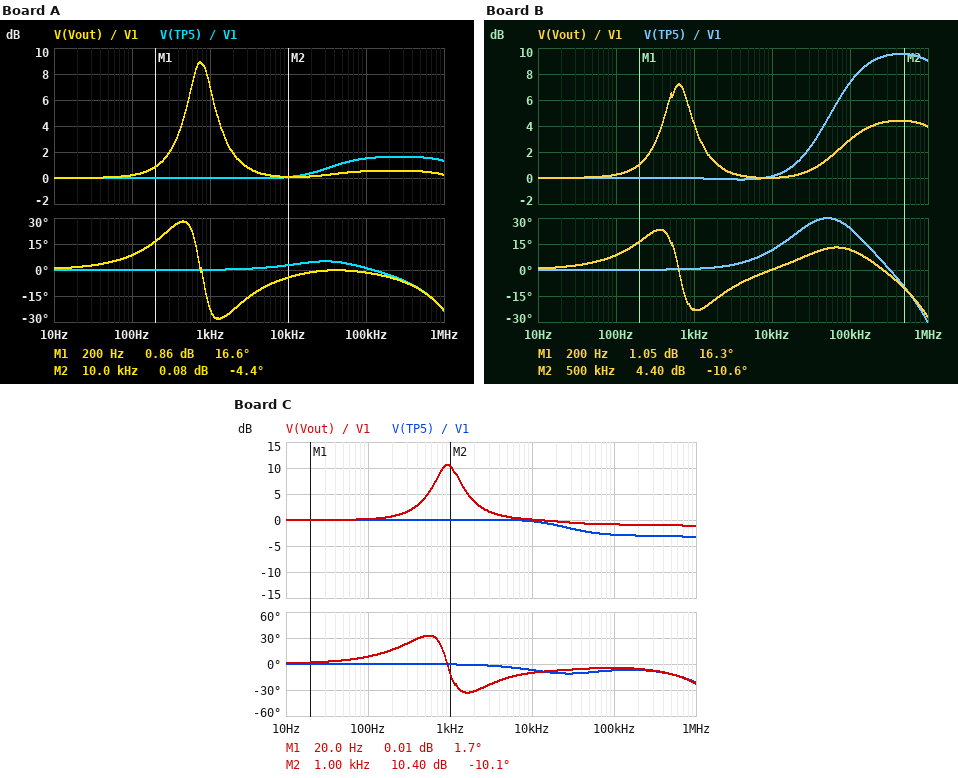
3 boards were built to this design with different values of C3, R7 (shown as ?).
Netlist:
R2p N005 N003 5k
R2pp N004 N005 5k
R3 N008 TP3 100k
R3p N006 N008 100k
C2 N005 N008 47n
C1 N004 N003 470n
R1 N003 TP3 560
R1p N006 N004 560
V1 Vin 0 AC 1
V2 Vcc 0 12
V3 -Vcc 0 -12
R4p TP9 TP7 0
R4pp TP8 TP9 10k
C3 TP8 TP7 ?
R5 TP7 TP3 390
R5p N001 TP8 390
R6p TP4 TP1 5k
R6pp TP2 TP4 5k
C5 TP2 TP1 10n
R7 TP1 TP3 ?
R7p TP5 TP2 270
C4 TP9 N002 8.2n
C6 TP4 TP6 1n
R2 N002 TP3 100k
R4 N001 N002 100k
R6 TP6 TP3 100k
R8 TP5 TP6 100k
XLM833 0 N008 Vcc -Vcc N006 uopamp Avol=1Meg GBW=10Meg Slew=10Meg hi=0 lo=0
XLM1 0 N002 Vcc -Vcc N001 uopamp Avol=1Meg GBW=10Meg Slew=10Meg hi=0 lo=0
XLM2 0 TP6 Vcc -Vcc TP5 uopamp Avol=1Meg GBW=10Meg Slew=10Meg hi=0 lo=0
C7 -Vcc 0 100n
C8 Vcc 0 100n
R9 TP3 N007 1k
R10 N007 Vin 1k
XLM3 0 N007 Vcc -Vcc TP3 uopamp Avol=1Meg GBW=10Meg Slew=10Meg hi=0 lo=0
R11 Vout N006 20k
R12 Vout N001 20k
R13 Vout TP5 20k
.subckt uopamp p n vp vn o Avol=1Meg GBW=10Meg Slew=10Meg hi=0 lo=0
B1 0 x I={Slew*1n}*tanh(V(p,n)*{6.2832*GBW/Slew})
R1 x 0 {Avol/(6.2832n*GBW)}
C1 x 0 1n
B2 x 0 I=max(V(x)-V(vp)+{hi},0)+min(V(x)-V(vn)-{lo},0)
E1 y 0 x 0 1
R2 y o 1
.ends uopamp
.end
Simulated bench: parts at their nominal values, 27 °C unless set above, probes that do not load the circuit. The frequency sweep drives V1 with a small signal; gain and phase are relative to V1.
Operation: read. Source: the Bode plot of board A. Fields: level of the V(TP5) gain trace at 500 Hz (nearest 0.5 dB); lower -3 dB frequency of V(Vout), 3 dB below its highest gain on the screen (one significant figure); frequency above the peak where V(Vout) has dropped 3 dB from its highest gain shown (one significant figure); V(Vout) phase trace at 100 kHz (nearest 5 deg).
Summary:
0 dB
500 Hz
1 kHz
0 deg
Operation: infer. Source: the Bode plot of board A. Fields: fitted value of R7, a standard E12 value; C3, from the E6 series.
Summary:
220 Ω
150 nF
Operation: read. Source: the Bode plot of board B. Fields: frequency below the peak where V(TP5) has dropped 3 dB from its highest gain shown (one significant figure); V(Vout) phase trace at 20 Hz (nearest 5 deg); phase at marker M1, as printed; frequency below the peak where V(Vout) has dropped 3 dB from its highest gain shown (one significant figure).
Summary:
80 kHz
0 deg
16.3 deg
400 Hz
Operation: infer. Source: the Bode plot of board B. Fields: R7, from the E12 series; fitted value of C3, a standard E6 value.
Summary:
82 Ω
220 nF
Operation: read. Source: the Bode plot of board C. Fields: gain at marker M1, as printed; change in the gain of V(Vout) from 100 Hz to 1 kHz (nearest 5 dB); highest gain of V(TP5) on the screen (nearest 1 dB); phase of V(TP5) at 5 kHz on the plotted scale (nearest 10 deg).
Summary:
0.01 dB
10 dB
0 dB
0 deg
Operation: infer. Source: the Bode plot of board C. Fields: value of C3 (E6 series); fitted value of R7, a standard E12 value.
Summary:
100 nF
390 Ω
